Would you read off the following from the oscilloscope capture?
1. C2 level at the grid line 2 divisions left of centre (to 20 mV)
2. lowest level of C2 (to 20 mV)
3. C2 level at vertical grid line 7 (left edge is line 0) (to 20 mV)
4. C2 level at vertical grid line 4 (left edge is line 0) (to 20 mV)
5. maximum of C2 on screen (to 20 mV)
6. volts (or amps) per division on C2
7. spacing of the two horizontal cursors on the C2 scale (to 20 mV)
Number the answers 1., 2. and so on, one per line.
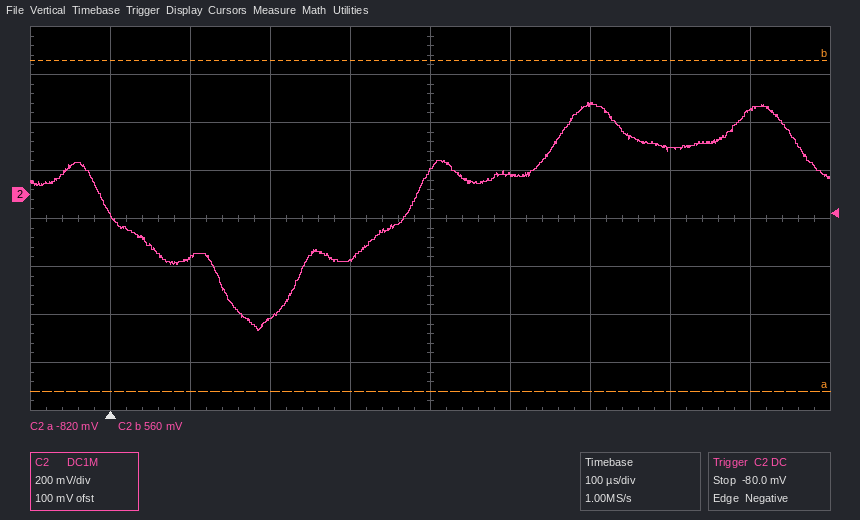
1. -520 mV
2. -560 mV
3. 380 mV
4. -260 mV
5. 380 mV
6. 200 mV
7. 1.38 V
